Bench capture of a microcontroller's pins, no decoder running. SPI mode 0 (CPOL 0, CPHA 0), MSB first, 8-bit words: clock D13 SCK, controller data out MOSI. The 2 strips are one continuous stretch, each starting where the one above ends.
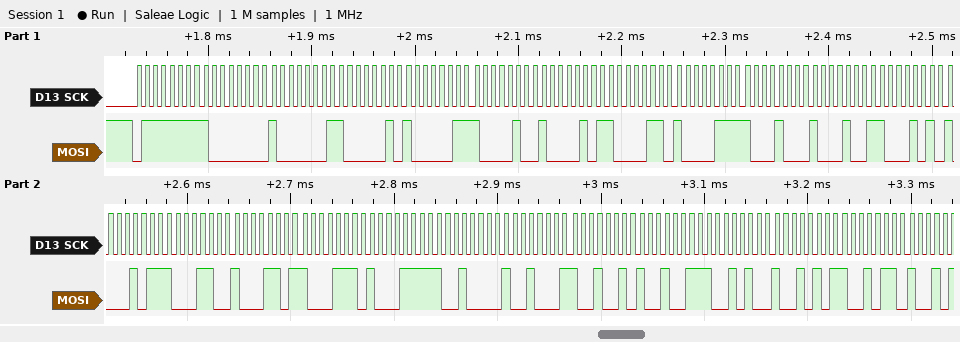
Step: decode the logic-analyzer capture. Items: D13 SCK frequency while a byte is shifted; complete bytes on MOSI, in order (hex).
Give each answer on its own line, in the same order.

125 kHz
0x7F 0x80 0x81 0x82 0x83 0x84 0x85 0x86 0x87 0x88 0x89 0x8A 0x8B 0x8C 0x8D 0x8E 0x8F 0x90 0x91 0x92 0x93 0x94 0x95 0x96
